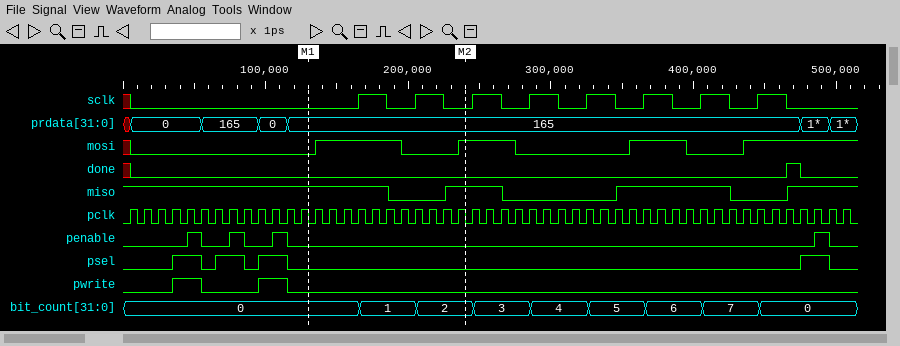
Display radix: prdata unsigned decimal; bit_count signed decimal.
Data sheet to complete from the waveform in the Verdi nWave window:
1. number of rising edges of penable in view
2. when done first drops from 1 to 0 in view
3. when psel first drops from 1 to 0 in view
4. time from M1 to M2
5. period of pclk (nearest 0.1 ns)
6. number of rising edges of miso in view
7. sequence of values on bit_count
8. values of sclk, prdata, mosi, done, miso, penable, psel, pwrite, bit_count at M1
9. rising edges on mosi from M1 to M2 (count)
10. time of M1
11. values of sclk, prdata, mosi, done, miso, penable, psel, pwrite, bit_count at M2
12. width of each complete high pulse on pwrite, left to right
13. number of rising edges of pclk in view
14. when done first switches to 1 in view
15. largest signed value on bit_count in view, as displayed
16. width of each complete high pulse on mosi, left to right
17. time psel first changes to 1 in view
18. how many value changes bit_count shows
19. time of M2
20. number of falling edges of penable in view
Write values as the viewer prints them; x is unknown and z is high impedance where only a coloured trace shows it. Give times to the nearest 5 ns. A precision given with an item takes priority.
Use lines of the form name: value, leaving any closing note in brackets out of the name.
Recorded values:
number of rising edges of penable in view: 4
when done first drops from 1 to 0 in view: 475 ns
when psel first drops from 1 to 0 in view: 55 ns
time from M1 to M2: 110 ns
period of pclk: 10 ns
number of rising edges of miso in view: 3
sequence of values on bit_count: 0, 1, 2, 3, 4, 5, 6, 7, 0
values of sclk, prdata, mosi, done, miso, penable, psel, pwrite, bit_count at M1: sclk=0, prdata=165, mosi=0, done=0, miso=1, penable=0, psel=0, pwrite=0, bit_count=0
rising edges on mosi from M1 to M2: 2
time of M1: 130 ns
values of sclk, prdata, mosi, done, miso, penable, psel, pwrite, bit_count at M2: sclk=0, prdata=165, mosi=1, done=0, miso=1, penable=0, psel=0, pwrite=0, bit_count=2
width of each complete high pulse on pwrite, left to right: 20 ns, 20 ns
number of rising edges of pclk in view: 51
when done first switches to 1 in view: 465 ns
largest signed value on bit_count in view, as displayed: 7
width of each complete high pulse on mosi, left to right: 60 ns, 40 ns, 40 ns
time psel first changes to 1 in view: 35 ns
how many value changes bit_count shows: 8
time of M2: 240 ns
number of falling edges of penable in view: 4
